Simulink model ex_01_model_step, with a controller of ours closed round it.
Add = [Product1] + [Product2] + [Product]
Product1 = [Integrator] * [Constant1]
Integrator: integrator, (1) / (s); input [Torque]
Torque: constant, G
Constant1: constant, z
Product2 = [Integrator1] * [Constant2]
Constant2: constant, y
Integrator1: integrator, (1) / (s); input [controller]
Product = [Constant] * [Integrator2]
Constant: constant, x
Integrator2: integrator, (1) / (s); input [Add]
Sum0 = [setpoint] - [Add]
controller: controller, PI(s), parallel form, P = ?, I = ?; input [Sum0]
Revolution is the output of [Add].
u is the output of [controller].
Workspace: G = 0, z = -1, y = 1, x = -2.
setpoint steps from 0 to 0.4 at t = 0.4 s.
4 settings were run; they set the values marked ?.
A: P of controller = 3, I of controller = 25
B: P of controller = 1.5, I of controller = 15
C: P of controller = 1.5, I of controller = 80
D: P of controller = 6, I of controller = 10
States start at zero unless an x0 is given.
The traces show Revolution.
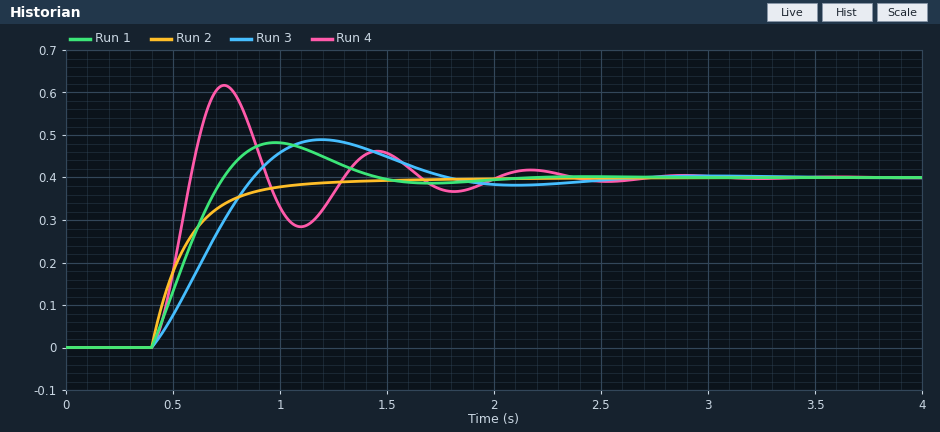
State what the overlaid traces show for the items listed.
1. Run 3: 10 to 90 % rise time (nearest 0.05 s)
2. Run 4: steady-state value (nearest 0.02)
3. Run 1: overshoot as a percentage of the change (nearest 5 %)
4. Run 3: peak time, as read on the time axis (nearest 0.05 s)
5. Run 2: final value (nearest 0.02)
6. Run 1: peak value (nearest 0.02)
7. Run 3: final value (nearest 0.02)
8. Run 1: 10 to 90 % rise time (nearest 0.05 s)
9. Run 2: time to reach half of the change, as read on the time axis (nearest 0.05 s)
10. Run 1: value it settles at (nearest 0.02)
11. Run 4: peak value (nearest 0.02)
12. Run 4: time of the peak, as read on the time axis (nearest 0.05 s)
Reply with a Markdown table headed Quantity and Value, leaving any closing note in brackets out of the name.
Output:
| Quantity | Value |
|---|---|
| Run 3: 10 to 90 % rise time | 0.35 s |
| Run 4: steady-state value | 0.40 |
| Run 1: overshoot as a percentage of the change | 20 % |
| Run 3: peak time, as read on the time axis | 1.20 s |
| Run 2: final value | 0.40 |
| Run 1: peak value | 0.48 |
| Run 3: final value | 0.40 |
| Run 1: 10 to 90 % rise time | 0.25 s |
| Run 2: time to reach half of the change, as read on the time axis | 0.50 s |
| Run 1: value it settles at | 0.40 |
| Run 4: peak value | 0.62 |
| Run 4: time of the peak, as read on the time axis | 0.75 s |
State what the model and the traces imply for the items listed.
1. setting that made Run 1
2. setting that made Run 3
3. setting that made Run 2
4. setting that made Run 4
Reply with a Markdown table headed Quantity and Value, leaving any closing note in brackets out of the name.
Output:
| Quantity | Value |
|---|---|
| setting that made Run 1 | A |
| setting that made Run 3 | B |
| setting that made Run 2 | D |
| setting that made Run 4 | C |
